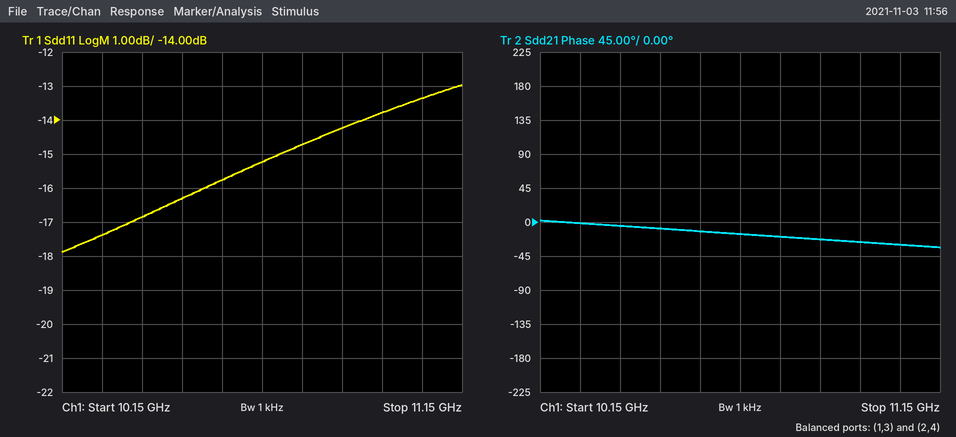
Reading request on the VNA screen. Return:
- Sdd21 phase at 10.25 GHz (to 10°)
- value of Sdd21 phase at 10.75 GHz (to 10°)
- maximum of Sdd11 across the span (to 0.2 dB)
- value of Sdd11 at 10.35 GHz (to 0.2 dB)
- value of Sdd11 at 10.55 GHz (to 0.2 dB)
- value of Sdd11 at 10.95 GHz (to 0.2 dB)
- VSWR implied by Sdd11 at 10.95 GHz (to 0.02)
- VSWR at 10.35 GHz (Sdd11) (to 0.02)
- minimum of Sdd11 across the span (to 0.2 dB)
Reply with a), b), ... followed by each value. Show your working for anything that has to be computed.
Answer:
a) 0°
b) -20°
c) -13.0 dB
d) -16.8 dB
e) -15.8 dB
f) -13.8 dB
g) |Γ| = 10^(-13.8/20) = 0.2042; VSWR = (1 + 0.2042)/(1 − 0.2042) ≈ 1.51, so 1.52 to the nearest 0.02
h) |Γ| = 10^(-16.8/20) = 0.1445; VSWR = (1 + 0.1445)/(1 − 0.1445) ≈ 1.34
i) -17.8 dB
